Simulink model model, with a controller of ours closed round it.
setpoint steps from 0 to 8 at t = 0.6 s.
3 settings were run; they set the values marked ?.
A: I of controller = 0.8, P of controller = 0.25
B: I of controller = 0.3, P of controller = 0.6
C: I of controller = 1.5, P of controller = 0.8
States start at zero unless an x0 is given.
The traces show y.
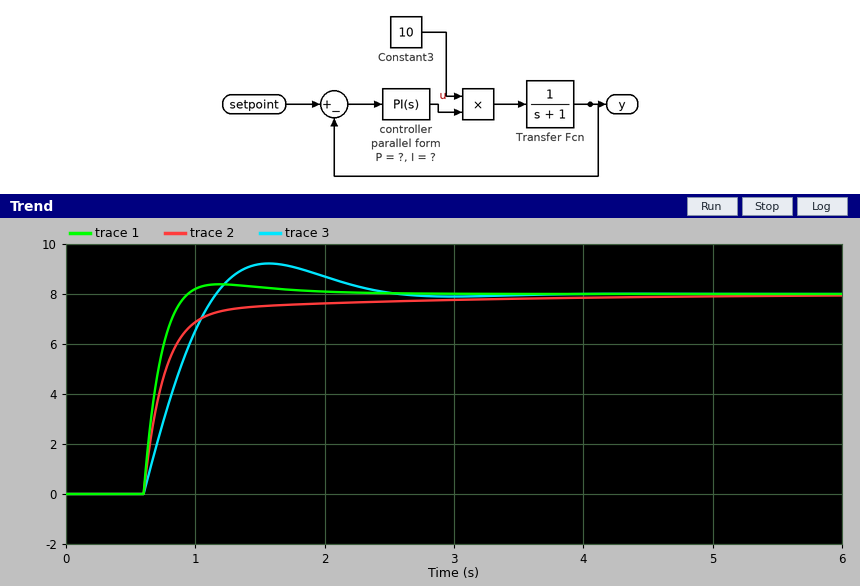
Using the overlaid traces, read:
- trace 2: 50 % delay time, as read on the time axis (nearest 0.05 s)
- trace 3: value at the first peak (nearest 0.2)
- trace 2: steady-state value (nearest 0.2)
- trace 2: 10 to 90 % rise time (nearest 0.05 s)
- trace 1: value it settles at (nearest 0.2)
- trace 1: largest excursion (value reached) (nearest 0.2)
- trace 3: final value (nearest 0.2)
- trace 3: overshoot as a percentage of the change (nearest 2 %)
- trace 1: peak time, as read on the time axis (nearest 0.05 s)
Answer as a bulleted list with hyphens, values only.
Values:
- 0.70 s
- 9.2
- 8.0
- 0.50 s
- 8.0
- 8.4
- 8.0
- 16 %
- 1.20 s
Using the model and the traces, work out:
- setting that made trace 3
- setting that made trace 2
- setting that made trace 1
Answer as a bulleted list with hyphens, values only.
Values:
- A
- B
- C
